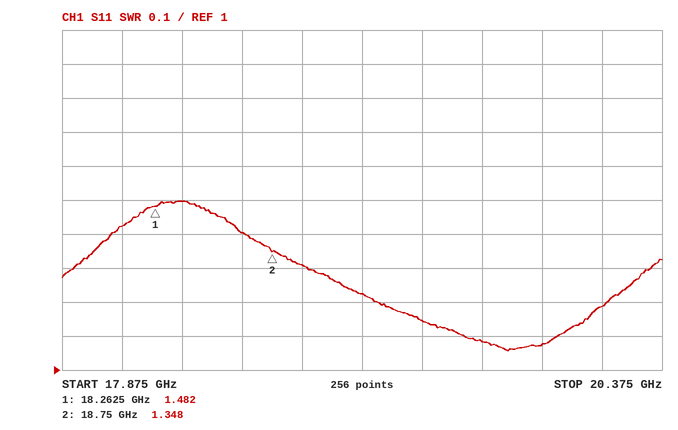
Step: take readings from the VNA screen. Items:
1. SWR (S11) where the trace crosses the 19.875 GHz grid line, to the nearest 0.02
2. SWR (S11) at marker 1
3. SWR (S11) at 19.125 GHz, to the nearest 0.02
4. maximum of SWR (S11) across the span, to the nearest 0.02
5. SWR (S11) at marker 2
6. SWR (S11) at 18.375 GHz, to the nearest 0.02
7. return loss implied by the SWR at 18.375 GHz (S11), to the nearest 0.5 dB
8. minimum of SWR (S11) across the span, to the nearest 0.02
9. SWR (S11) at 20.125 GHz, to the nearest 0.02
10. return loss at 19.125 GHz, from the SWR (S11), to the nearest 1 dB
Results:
1.08
1.482
1.22
1.50
1.348
1.50
14.0 dB
1.06
1.18
20 dB
